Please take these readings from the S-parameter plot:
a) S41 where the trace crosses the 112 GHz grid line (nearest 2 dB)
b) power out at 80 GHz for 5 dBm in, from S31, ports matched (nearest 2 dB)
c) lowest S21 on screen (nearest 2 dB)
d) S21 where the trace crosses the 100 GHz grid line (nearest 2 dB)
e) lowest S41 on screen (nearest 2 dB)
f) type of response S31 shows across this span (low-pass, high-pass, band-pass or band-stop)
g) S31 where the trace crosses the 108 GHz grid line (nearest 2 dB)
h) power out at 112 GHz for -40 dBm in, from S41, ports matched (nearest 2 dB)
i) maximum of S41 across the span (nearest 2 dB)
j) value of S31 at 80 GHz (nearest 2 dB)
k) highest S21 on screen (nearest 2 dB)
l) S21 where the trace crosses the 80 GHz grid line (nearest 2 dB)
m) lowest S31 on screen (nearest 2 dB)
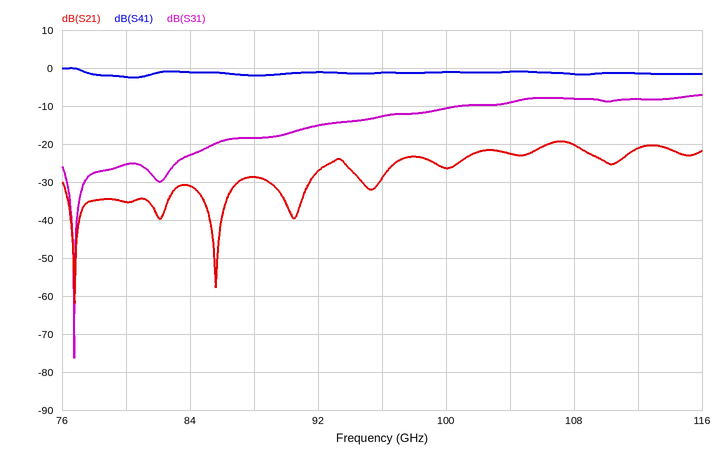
-2 dB
-20 dBm
-62 dB
-26 dB
-2 dB
high-pass
-8 dB
-42 dBm
0 dB
-26 dB
-20 dB
-36 dB
-76 dB
